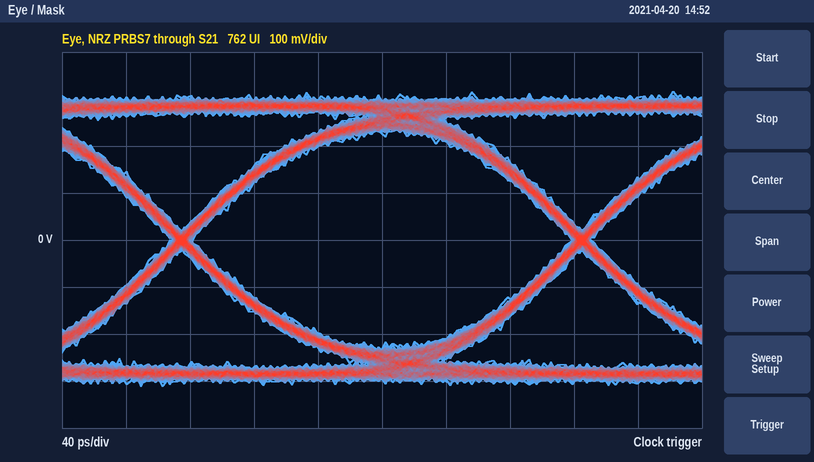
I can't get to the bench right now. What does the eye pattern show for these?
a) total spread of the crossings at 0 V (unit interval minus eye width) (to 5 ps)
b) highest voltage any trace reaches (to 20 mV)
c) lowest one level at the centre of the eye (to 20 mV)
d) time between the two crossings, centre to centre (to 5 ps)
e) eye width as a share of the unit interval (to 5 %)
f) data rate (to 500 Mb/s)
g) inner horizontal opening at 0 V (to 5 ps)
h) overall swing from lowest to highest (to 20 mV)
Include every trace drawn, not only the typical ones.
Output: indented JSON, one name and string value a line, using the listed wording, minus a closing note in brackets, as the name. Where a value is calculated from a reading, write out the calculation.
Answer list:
{
  "total spread of the crossings at 0 V (unit interval minus eye width)": "15 ps",
  "highest voltage any trace reaches": "320 mV",
  "lowest one level at the centre of the eye": "220 mV",
  "time between the two crossings, centre to centre": "250 ps",
  "eye width as a share of the unit interval": "235 ps / 250 ps ≈ 94.0 %, so 95 % to the nearest 5 %",
  "data rate": "4.0 Gb/s",
  "inner horizontal opening at 0 V": "235 ps",
  "overall swing from lowest to highest": "620 mV"
}
